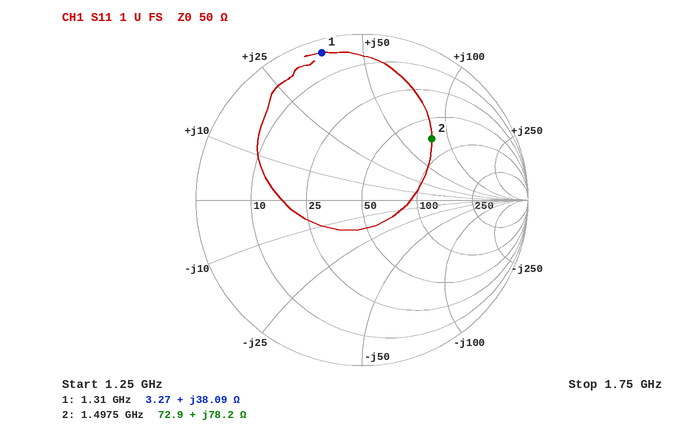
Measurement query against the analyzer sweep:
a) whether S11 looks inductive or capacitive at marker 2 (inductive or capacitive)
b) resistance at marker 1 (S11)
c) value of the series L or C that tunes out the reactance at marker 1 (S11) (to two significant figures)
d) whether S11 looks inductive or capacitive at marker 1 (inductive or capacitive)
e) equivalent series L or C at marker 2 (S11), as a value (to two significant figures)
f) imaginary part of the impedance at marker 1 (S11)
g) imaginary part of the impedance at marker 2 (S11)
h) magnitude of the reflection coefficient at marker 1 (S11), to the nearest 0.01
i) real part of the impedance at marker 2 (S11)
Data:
inductive
3.27 Ω
3.2 pF
inductive
8.3 nH
+38.09 Ω
+78.2 Ω
0.92
72.9 Ω
